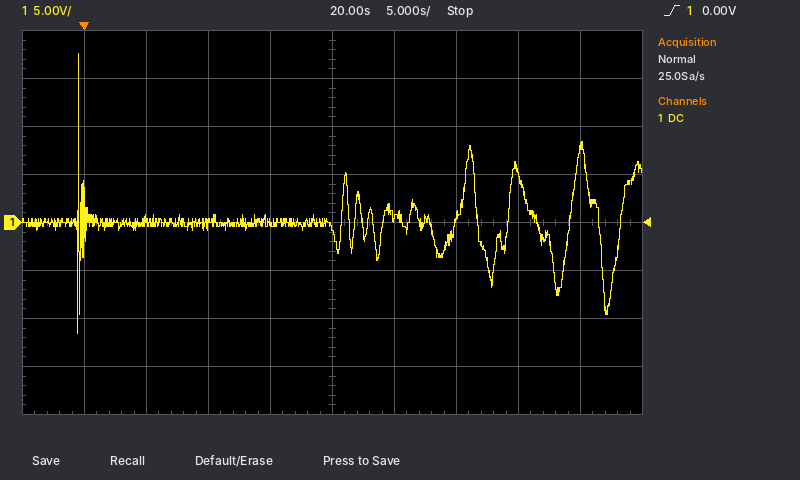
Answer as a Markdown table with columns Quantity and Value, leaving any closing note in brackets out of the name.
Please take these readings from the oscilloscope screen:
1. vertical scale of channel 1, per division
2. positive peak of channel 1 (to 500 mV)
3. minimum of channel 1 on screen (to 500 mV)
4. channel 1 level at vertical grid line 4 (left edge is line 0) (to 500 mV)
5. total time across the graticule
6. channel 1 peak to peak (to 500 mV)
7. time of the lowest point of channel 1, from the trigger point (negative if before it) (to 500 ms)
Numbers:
| Quantity | Value |
|---|---|
| vertical scale of channel 1, per division | 5 V |
| positive peak of channel 1 | 17.5 V |
| minimum of channel 1 on screen | -11.5 V |
| channel 1 level at vertical grid line 4 (left edge is line 0) | 0.0 V |
| total time across the graticule | 50 s |
| channel 1 peak to peak | 29.0 V |
| time of the lowest point of channel 1, from the trigger point (negative if before it) | -500 ms |
